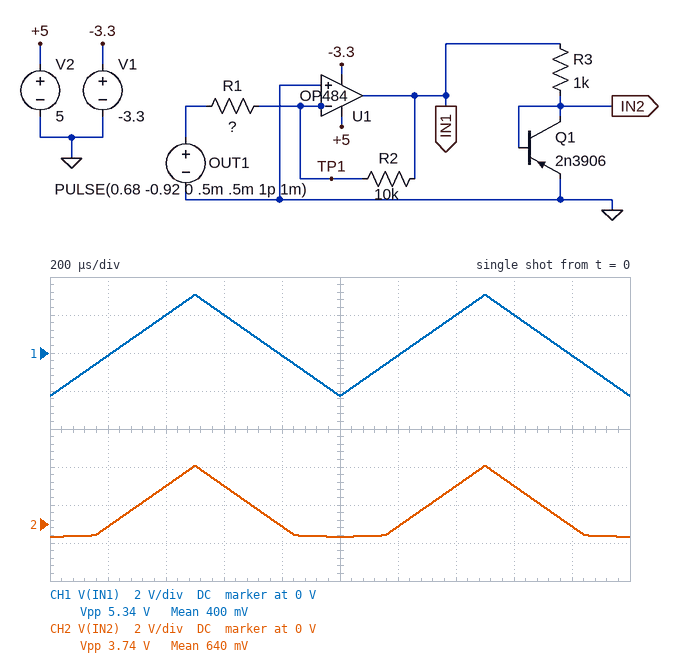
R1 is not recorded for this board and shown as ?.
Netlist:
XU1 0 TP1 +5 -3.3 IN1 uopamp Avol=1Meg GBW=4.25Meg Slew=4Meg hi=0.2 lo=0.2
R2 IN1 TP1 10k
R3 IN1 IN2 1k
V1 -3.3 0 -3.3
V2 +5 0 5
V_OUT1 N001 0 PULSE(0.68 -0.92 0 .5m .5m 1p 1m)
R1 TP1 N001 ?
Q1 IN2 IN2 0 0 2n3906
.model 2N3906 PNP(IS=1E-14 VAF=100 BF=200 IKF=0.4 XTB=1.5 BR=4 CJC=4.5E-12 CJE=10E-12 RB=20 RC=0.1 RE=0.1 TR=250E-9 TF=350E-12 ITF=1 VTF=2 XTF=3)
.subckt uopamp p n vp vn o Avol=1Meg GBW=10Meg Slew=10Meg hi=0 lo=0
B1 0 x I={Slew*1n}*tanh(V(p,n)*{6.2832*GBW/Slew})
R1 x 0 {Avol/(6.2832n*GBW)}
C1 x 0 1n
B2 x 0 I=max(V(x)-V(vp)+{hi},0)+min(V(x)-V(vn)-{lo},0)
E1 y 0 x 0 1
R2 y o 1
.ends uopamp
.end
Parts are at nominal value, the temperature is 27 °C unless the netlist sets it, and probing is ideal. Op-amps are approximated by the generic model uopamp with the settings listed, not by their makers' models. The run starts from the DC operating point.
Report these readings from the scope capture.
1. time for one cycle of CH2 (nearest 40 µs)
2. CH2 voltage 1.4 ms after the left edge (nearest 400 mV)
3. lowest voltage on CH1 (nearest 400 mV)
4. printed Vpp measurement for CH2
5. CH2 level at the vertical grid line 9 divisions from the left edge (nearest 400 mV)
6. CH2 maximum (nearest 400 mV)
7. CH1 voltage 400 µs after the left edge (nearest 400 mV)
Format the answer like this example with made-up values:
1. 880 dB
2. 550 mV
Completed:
1. 1.00 ms
2. 2.0 V
3. -2.4 V
4. 3.74 V
5. 0 V
6. 3.2 V
7. 2.0 V
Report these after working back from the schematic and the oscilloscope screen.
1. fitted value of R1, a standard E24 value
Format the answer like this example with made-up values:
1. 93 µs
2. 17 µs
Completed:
1. 3 kΩ
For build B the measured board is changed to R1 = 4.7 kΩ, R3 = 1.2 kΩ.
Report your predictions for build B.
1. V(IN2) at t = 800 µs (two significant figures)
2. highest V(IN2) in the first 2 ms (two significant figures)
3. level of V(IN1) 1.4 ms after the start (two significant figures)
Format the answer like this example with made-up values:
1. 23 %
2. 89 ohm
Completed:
1. -84 mV
2. 2.0 V
3. 1.3 V
